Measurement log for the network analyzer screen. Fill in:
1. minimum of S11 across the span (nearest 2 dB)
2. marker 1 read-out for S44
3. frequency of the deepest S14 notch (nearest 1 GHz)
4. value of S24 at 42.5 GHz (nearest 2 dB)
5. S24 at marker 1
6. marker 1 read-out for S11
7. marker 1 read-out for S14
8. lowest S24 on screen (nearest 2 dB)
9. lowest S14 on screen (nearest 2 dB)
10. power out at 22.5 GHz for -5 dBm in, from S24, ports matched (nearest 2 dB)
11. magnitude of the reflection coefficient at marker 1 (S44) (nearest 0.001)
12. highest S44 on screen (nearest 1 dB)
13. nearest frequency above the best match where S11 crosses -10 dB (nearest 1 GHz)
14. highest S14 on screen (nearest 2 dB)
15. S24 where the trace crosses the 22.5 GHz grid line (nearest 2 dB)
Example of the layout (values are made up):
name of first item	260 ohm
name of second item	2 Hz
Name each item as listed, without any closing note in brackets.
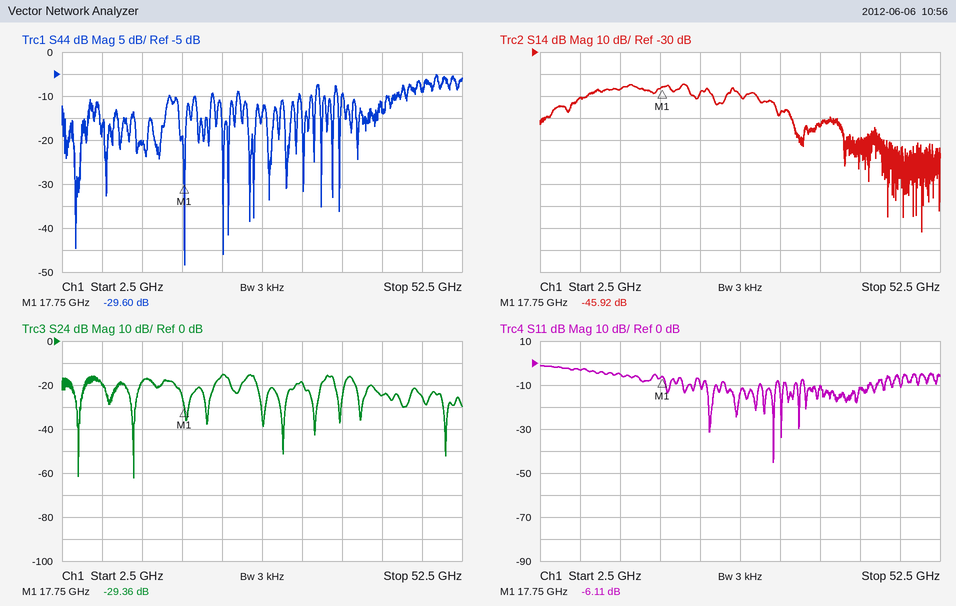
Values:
minimum of S11 across the span	-46 dB
marker 1 read-out for S44	-29.60 dB
frequency of the deepest S14 notch	50 GHz
value of S24 at 42.5 GHz	-24 dB
S24 at marker 1	-29.36 dB
marker 1 read-out for S11	-6.11 dB
marker 1 read-out for S14	-45.92 dB
lowest S24 on screen	-62 dB
lowest S14 on screen	-112 dB
power out at 22.5 GHz for -5 dBm in, from S24, ports matched	-20 dBm
magnitude of the reflection coefficient at marker 1 (S44)	0.033
highest S44 on screen	-5 dB
nearest frequency above the best match where S11 crosses -10 dB	32 GHz
highest S14 on screen	-44 dB
S24 where the trace crosses the 22.5 GHz grid line	-16 dB
